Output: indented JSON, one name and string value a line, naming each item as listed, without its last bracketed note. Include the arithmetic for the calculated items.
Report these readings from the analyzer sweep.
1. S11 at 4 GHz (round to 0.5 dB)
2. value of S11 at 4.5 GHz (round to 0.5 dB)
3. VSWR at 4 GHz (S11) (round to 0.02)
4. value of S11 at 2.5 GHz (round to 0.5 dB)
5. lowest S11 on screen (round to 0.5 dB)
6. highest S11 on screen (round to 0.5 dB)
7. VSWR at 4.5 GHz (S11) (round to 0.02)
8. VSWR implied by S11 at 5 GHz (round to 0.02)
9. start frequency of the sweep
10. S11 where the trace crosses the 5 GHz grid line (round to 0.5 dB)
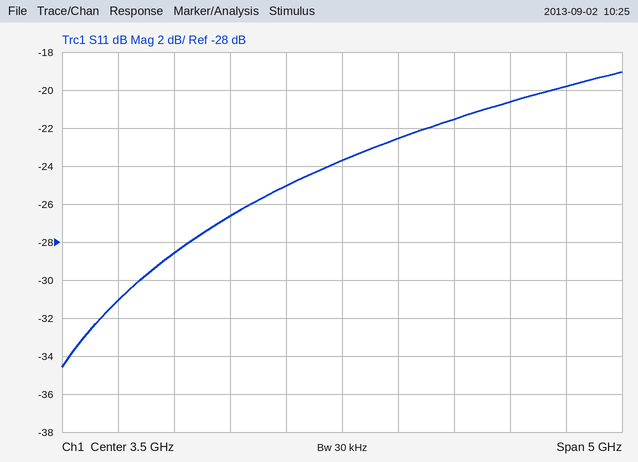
{
  "S11 at 4 GHz": "-22.5 dB",
  "value of S11 at 4.5 GHz": "-21.5 dB",
  "VSWR at 4 GHz (S11)": "|Γ| = 10^(-22.5/20) = 0.0750; VSWR = (1 + 0.0750)/(1 − 0.0750) ≈ 1.16",
  "value of S11 at 2.5 GHz": "-26.5 dB",
  "lowest S11 on screen": "-34.5 dB",
  "highest S11 on screen": "-19.0 dB",
  "VSWR at 4.5 GHz (S11)": "|Γ| = 10^(-21.5/20) = 0.0841; VSWR = (1 + 0.0841)/(1 − 0.0841) ≈ 1.18",
  "VSWR implied by S11 at 5 GHz": "|Γ| = 10^(-20.5/20) = 0.0944; VSWR = (1 + 0.0944)/(1 − 0.0944) ≈ 1.21, so 1.20 to the nearest 0.02",
  "start frequency of the sweep": "1 GHz",
  "S11 where the trace crosses the 5 GHz grid line": "-20.5 dB"
}
